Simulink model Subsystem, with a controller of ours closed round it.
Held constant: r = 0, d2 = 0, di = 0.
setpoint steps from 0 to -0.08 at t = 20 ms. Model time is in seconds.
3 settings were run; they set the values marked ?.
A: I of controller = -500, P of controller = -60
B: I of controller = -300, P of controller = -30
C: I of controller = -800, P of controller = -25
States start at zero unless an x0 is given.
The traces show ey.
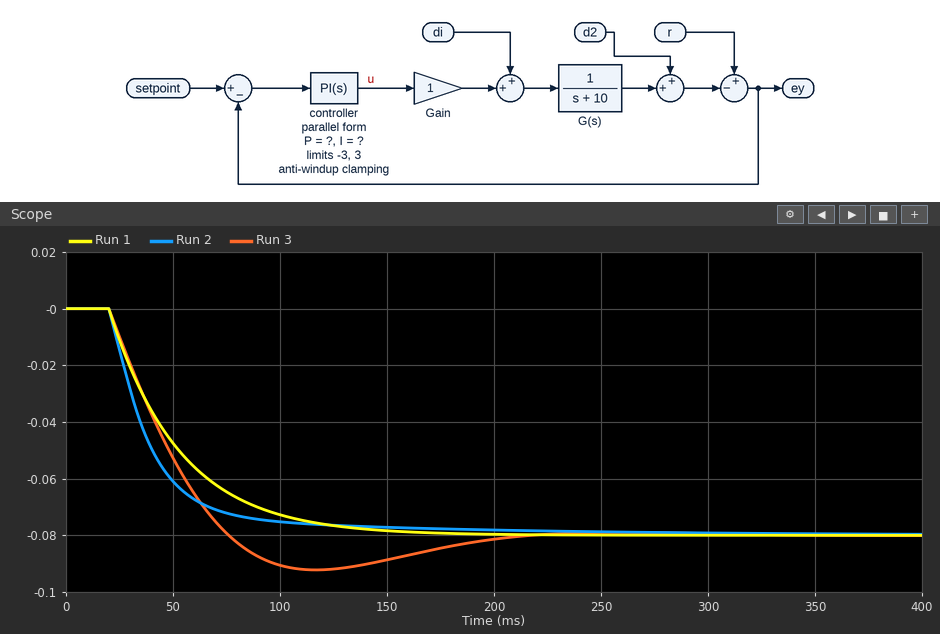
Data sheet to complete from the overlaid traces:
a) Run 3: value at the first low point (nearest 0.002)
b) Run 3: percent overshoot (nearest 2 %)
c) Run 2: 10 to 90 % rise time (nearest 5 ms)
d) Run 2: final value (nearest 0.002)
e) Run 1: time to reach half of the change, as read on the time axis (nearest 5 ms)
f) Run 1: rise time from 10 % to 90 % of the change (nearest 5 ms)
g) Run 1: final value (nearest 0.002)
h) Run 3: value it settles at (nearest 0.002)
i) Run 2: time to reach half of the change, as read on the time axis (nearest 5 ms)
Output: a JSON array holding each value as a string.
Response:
["-0.092", "16 %", "50 ms", "-0.080", "45 ms", "75 ms", "-0.080", "-0.080", "35 ms"]
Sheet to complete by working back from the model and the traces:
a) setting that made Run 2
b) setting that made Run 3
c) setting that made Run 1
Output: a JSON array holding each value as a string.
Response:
["A", "C", "B"]
